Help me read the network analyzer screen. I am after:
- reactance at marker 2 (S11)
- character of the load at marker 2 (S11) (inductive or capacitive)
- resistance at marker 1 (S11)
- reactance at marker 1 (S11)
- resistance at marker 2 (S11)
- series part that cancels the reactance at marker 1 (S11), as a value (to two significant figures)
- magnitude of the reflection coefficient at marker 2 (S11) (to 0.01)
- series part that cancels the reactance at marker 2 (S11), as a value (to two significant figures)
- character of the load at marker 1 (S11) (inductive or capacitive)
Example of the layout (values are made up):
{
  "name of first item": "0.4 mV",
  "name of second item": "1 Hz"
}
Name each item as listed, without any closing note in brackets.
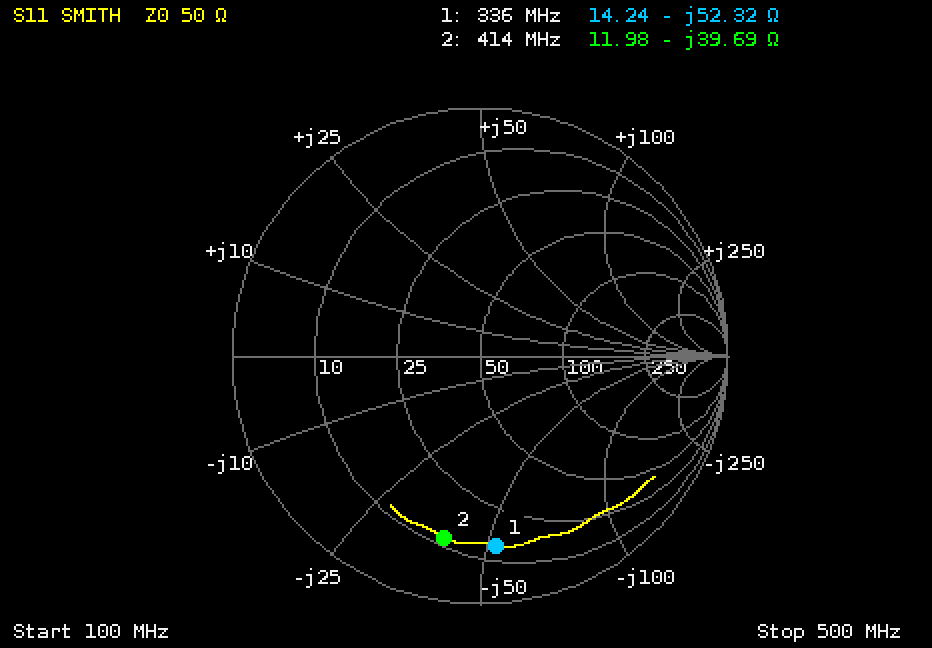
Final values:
{
  "reactance at marker 2": "-39.69 Ω",
  "character of the load at marker 2 (S11)": "capacitive",
  "resistance at marker 1": "14.24 Ω",
  "reactance at marker 1": "-52.32 Ω",
  "resistance at marker 2": "11.98 Ω",
  "series part that cancels the reactance at marker 1 (S11), as a value": "25 nH",
  "magnitude of the reflection coefficient at marker 2 (S11)": "0.75",
  "series part that cancels the reactance at marker 2 (S11), as a value": "15 nH",
  "character of the load at marker 1 (S11)": "capacitive"
}
